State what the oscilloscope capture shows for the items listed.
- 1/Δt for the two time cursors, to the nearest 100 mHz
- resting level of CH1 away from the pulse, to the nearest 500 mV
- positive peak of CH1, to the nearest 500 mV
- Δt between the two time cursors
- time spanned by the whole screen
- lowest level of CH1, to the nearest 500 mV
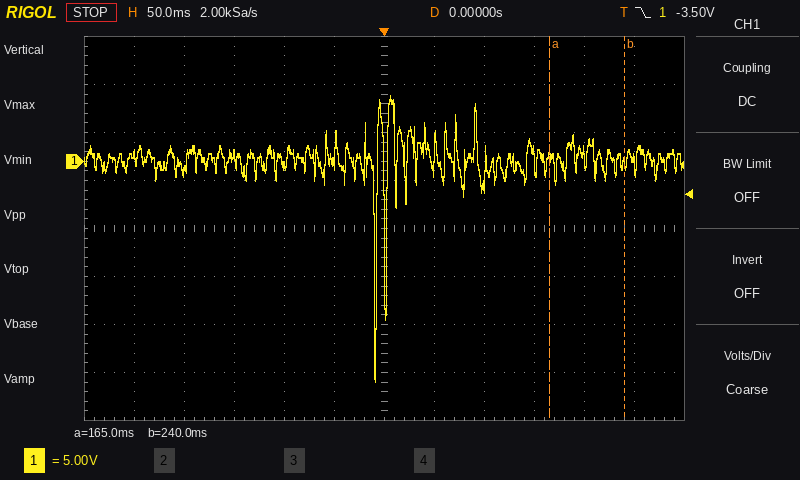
13.3 Hz
500 mV
7.0 V
75 ms
600 ms
-23.0 V
